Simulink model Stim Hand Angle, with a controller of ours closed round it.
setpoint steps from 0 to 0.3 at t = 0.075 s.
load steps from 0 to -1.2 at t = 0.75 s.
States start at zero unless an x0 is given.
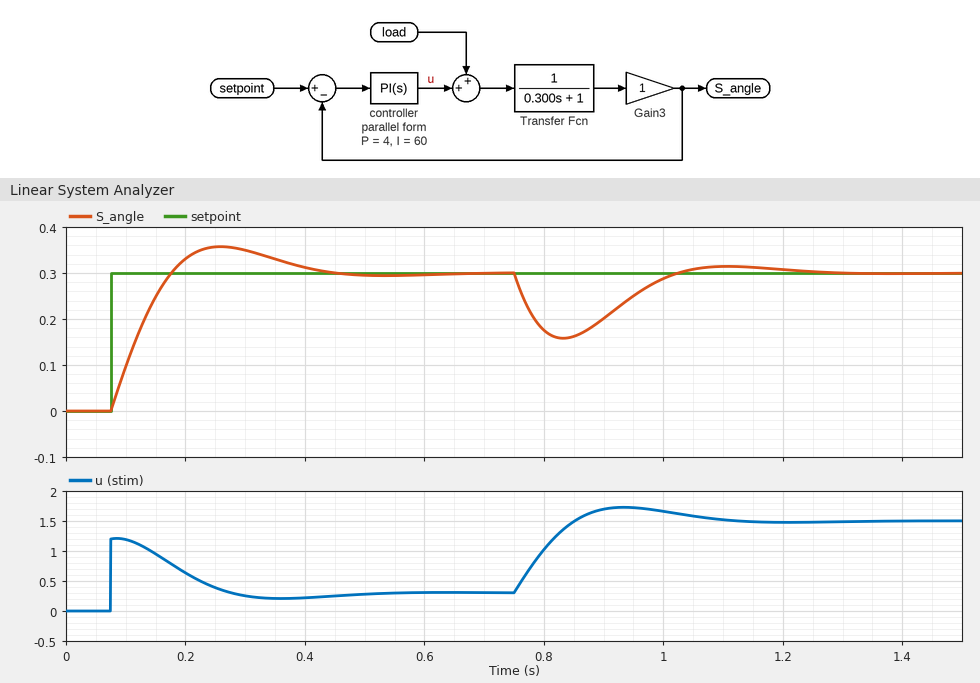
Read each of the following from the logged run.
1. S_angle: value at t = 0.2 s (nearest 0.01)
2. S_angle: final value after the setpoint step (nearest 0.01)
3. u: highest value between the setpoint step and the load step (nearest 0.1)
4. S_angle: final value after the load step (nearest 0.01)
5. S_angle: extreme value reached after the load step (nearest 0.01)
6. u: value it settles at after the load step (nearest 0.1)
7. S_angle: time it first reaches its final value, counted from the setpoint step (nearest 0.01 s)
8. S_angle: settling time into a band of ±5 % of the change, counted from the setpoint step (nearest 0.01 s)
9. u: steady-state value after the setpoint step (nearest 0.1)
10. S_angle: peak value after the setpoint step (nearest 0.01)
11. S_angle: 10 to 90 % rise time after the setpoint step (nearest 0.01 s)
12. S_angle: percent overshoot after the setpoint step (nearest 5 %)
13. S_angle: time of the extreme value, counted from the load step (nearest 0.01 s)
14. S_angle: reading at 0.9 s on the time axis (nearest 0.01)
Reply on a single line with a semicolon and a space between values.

0.33; 0.30; 1.2; 0.30; 0.16; 1.5; 0.10 s; 0.32 s; 0.3; 0.36; 0.08 s; 20 %; 0.08 s; 0.20
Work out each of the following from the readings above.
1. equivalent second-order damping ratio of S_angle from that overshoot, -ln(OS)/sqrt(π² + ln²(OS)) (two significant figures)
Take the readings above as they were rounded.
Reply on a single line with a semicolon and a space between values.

0.46
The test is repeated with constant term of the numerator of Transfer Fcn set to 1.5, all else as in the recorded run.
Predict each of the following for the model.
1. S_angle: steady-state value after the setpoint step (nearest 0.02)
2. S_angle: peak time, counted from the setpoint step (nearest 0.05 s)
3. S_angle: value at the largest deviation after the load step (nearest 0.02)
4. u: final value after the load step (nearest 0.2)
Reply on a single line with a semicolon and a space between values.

0.30; 0.15 s; 0.14; 1.4
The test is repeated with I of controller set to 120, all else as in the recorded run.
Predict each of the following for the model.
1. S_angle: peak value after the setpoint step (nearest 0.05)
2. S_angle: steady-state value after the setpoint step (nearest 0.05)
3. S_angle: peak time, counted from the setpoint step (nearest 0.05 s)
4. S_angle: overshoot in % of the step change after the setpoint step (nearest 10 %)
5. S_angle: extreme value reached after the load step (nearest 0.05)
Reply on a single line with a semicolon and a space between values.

0.40; 0.30; 0.15 s; 30 %; 0.20
